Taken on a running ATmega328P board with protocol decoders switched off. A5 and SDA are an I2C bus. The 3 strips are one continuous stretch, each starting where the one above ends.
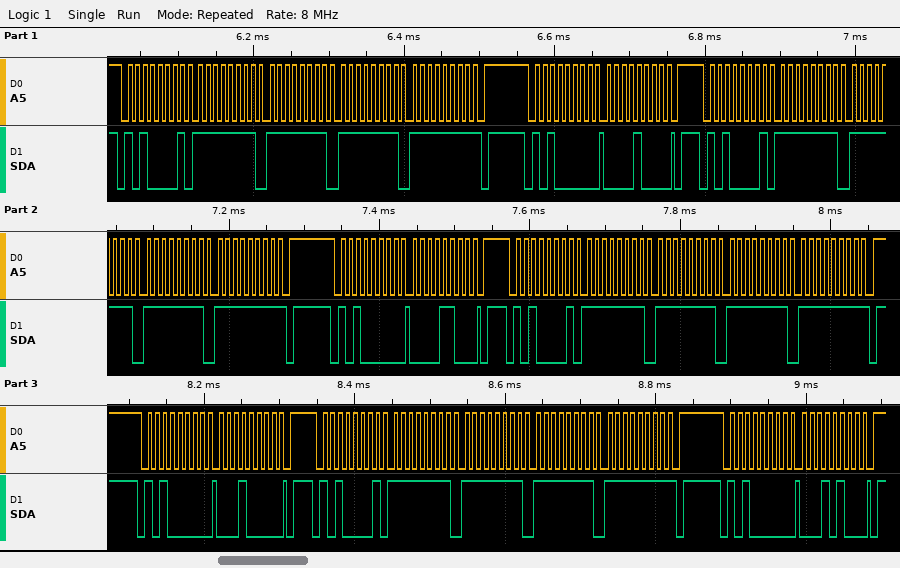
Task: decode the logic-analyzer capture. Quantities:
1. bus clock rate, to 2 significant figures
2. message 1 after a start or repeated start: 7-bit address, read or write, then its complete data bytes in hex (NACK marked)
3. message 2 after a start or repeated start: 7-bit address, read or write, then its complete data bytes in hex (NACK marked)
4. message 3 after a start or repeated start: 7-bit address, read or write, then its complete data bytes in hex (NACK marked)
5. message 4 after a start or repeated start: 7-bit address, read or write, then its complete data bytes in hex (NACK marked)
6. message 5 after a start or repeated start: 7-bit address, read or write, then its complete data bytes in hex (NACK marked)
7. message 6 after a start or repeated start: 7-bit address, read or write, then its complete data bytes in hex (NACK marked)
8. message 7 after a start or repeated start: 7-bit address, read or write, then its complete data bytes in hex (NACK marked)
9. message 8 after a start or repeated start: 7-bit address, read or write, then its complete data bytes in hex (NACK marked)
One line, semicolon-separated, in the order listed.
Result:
100 kHz; 0x50 read: FF FF FF FF NACK; 0x50 write: 08; 0x50 read: FF FF FF FF NACK; 0x50 write: 0C; 0x50 read: FF FF FF FF NACK; 0x50 write: 10; 0x50 read: FF FF FF FF NACK; 0x50 write: 14
